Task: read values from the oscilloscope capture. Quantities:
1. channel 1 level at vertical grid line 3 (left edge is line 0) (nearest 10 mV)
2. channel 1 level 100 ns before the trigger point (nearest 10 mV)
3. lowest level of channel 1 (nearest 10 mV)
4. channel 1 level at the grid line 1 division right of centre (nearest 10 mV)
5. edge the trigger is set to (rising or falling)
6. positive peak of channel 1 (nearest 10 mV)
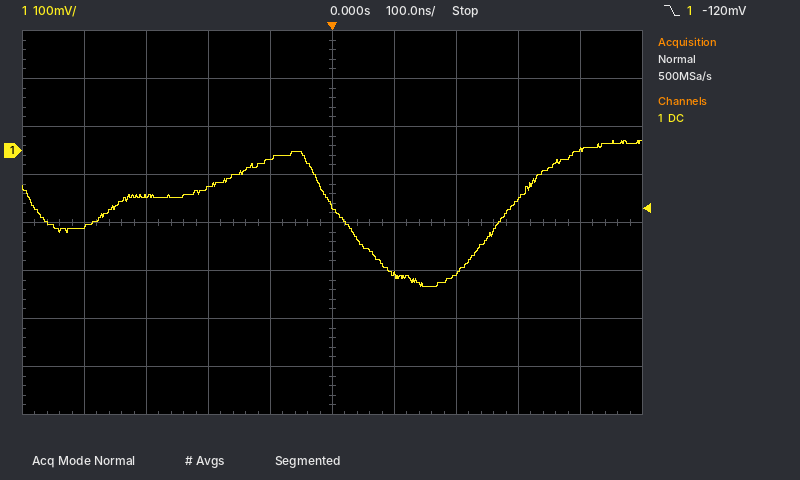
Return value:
-80 mV
-20 mV
-280 mV
-260 mV
falling
20 mV
